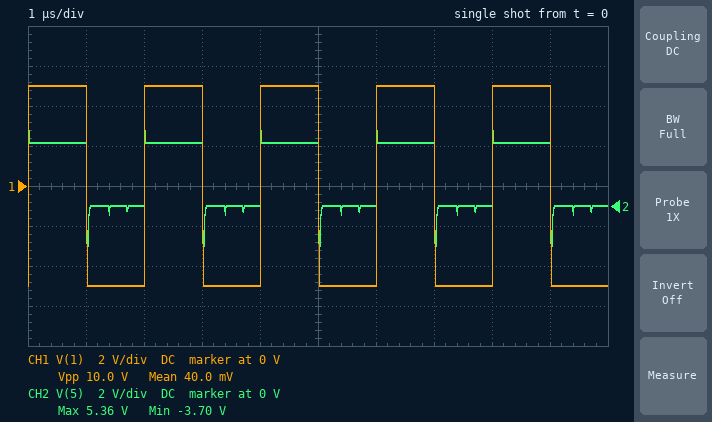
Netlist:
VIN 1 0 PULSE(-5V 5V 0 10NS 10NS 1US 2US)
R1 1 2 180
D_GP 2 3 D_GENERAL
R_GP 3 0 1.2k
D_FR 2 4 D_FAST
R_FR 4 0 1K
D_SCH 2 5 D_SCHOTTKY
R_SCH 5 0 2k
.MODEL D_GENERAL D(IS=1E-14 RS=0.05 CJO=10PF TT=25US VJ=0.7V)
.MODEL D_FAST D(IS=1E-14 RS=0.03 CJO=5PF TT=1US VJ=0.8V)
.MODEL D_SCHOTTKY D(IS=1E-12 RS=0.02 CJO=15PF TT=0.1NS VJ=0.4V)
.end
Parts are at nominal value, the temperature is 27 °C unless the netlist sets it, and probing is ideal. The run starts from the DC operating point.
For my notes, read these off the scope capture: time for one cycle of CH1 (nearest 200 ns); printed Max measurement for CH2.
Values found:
2.0 µs
5.36 V
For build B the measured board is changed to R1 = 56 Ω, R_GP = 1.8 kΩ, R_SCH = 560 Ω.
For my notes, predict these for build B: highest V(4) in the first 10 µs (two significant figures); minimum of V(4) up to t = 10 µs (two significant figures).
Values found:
3.7 V
-5.2 V
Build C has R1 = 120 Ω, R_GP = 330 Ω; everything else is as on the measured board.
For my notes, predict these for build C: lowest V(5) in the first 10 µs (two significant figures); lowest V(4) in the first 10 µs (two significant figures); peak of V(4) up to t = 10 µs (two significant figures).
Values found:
-3.4 V
-3.8 V
2.9 V
